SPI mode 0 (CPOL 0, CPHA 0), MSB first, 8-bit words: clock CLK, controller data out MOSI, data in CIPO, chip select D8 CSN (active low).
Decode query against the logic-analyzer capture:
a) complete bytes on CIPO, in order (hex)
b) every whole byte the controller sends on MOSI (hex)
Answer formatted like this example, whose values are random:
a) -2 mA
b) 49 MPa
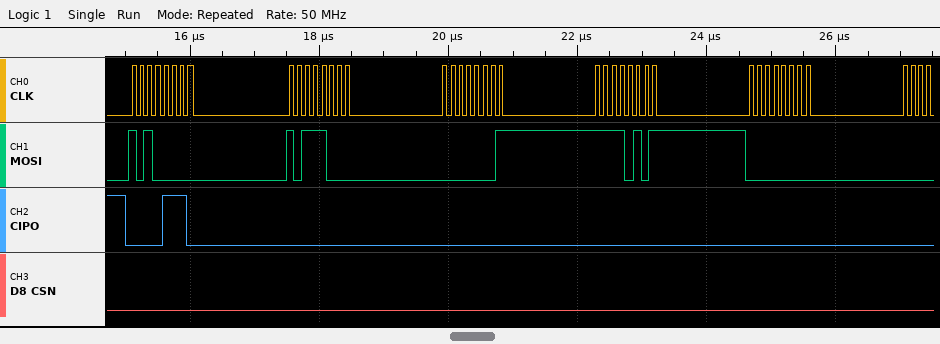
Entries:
a) 0E 00 00 00 00
b) A0 B8 01 F5 00
